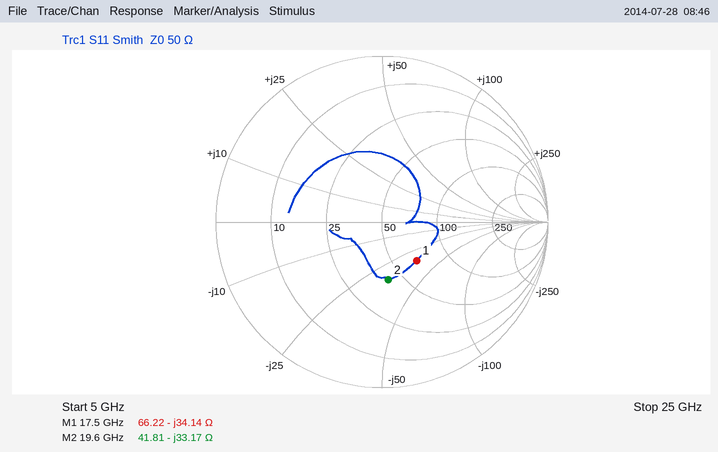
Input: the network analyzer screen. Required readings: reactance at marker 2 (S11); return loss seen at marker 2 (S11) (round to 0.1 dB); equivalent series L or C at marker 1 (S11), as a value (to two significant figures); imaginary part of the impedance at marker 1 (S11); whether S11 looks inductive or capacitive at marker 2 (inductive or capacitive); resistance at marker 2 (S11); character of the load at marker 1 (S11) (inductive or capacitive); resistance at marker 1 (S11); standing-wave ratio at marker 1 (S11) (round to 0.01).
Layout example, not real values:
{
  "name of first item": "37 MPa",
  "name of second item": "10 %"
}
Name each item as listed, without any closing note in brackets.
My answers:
{
  "reactance at marker 2": "-33.17 Ω",
  "return loss seen at marker 2 (S11)": "9.1 dB",
  "equivalent series L or C at marker 1 (S11), as a value": "270 fF",
  "imaginary part of the impedance at marker 1": "-34.14 Ω",
  "whether S11 looks inductive or capacitive at marker 2": "capacitive",
  "resistance at marker 2": "41.81 Ω",
  "character of the load at marker 1 (S11)": "capacitive",
  "resistance at marker 1": "66.22 Ω",
  "standing-wave ratio at marker 1 (S11)": "1.91"
}
